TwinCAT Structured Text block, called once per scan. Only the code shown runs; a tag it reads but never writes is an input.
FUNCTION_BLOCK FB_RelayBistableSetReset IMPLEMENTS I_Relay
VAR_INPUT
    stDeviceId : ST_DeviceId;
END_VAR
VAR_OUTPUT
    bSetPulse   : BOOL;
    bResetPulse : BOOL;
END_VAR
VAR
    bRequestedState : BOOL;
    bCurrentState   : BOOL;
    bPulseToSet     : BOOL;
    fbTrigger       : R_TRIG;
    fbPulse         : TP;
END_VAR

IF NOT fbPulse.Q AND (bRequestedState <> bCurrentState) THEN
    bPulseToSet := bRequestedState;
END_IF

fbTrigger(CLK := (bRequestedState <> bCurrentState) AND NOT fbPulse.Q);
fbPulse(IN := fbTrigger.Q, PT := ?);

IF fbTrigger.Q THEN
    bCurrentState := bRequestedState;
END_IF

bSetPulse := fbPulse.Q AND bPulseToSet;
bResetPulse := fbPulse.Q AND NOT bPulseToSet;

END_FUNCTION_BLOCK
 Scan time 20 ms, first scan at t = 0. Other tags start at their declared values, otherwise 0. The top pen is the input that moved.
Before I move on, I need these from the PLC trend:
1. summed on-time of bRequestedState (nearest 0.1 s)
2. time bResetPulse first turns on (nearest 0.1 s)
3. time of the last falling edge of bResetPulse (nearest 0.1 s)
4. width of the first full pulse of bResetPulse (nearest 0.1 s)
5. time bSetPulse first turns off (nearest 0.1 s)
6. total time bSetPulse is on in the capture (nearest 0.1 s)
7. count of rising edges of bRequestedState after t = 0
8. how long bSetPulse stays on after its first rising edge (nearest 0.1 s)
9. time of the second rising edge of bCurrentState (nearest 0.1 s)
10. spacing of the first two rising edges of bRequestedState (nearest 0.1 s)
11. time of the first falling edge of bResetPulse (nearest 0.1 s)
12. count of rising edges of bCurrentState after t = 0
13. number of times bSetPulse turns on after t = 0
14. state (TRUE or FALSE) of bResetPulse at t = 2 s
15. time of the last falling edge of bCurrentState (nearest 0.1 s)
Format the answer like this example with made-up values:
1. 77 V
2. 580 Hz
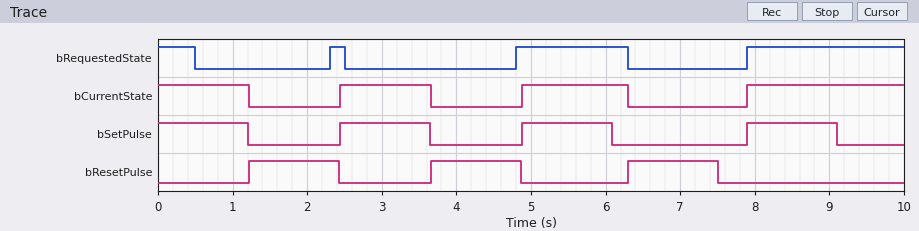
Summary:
1. 4.3 s
2. 1.2 s
3. 7.5 s
4. 1.2 s
5. 1.2 s
6. 4.8 s
7. 3
8. 1.2 s
9. 4.9 s
10. 2.5 s
11. 2.4 s
12. 3
13. 3
14. TRUE
15. 6.3 s
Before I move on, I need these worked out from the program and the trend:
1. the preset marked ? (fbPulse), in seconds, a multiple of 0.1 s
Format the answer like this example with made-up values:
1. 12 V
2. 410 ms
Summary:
1. 1.2 s
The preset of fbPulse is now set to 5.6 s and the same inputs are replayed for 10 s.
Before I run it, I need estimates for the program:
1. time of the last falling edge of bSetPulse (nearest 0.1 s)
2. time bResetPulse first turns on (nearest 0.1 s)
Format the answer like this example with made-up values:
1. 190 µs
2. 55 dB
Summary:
1. 5.6 s
2. 6.3 s
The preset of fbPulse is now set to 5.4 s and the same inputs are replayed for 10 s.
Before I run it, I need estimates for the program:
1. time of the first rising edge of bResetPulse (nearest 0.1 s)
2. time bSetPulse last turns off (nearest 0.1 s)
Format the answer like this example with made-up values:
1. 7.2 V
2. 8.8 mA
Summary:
1. 6.3 s
2. 5.4 s
